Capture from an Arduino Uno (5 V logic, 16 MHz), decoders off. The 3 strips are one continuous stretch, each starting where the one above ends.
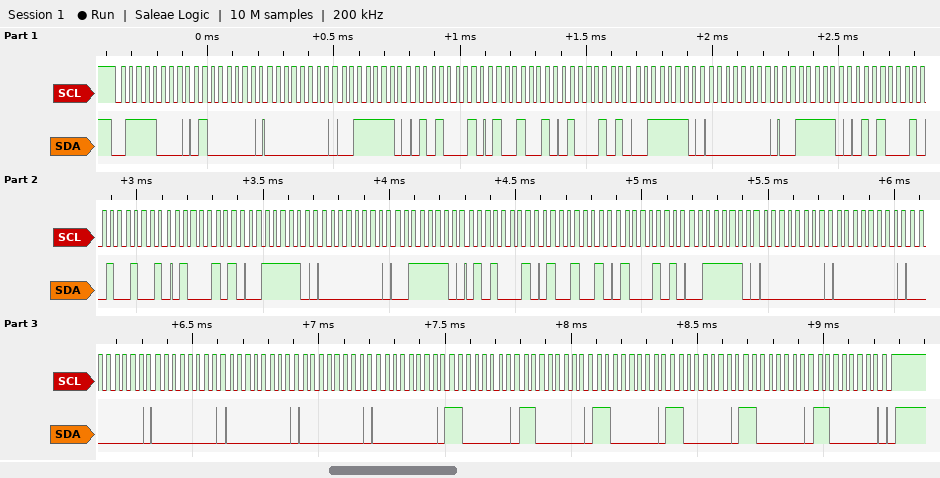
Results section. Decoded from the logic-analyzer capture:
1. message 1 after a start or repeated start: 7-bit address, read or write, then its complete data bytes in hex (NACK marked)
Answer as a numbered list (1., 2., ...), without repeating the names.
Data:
1. 0x3C write: 40 00 3E 51 49 45 3E 00 3E 51 49 45 3E 00 3E 51 49 45 3E 00 00 00 00 00 00 00 C0 C0 C0 C0 C0 C0
